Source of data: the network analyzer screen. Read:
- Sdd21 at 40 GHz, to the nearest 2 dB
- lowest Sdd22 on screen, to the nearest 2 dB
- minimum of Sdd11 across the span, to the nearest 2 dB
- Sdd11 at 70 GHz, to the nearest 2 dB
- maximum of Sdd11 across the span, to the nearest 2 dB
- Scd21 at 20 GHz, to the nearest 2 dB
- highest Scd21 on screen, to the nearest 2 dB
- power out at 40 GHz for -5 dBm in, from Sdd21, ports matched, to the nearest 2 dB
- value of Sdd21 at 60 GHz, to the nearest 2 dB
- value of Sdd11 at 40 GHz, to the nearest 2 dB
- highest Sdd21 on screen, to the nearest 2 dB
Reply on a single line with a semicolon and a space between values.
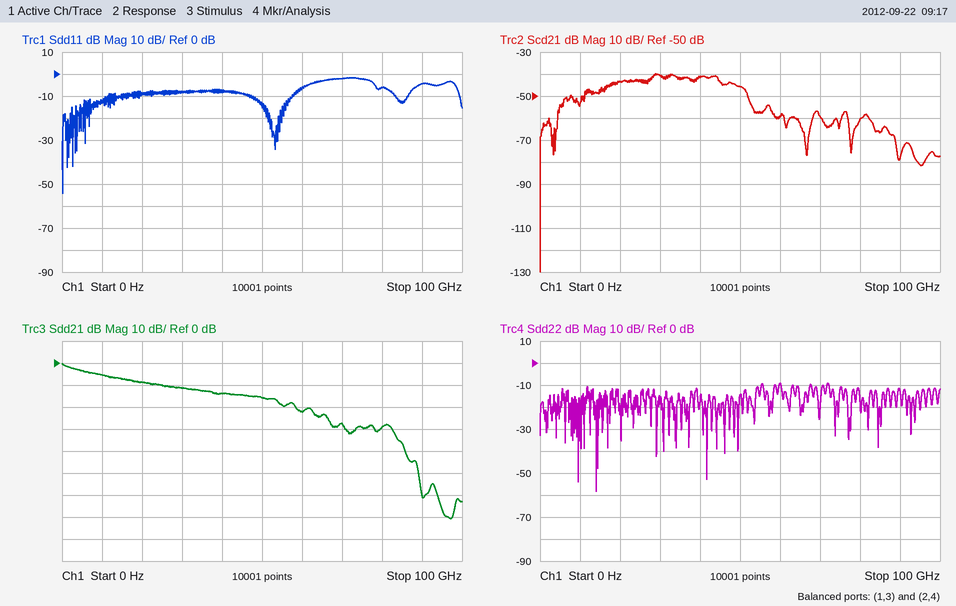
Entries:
-14 dB; -58 dB; -54 dB; -2 dB; -2 dB; -44 dB; -40 dB; -18 dBm; -22 dB; -8 dB; 0 dB
